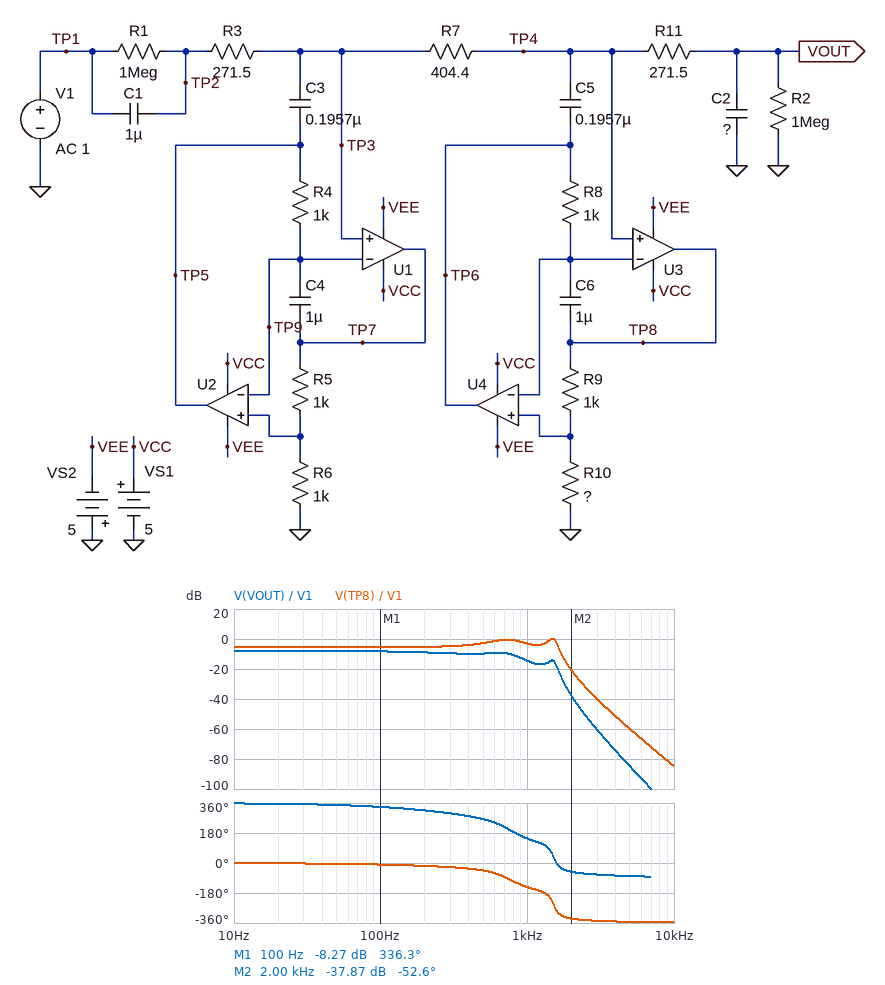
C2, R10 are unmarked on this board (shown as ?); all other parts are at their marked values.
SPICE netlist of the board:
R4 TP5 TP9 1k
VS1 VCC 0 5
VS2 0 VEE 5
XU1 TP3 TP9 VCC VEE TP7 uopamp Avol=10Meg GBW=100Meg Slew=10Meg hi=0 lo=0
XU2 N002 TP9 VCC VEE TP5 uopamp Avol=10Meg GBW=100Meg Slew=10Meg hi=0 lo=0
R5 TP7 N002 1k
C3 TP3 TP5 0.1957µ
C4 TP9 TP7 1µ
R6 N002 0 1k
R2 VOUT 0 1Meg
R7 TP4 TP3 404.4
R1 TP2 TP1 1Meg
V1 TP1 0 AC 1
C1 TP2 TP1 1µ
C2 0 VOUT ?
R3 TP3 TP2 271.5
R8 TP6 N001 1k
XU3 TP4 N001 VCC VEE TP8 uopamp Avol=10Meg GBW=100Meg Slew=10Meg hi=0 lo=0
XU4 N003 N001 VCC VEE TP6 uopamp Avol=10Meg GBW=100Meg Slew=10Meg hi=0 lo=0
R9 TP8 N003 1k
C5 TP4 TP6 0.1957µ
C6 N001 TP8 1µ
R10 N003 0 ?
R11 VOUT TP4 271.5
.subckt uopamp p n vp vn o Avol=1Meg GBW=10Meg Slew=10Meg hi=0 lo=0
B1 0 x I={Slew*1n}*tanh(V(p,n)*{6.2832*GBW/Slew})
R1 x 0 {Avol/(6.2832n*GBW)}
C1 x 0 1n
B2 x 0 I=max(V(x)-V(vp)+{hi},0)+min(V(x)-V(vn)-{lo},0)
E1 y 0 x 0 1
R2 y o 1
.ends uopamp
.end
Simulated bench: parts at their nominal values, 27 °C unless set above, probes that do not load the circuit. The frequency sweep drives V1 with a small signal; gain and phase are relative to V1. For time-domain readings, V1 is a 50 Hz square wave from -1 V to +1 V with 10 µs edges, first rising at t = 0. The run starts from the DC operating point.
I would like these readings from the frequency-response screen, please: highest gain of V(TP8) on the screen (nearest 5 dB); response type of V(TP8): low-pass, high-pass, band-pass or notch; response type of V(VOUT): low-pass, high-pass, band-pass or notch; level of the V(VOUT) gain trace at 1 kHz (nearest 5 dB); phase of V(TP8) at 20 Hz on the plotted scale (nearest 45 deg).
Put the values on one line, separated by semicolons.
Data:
0 dB; low-pass; low-pass; -15 dB; 0 deg
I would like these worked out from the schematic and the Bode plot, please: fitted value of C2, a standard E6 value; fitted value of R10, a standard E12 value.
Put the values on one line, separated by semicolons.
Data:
1.5 µF; 2.7 kΩ
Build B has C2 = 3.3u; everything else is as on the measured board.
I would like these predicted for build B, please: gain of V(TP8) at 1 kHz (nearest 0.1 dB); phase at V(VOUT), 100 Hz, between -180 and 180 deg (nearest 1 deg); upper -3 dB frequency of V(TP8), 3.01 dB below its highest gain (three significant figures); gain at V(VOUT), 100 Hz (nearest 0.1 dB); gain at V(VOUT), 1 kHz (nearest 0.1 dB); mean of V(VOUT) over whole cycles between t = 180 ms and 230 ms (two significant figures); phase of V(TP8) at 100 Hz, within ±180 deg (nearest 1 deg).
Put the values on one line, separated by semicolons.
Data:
-3.2 dB; -27 deg; 1.56 kHz; -13.2 dB; -21.1 dB; -240 mV; 2 deg
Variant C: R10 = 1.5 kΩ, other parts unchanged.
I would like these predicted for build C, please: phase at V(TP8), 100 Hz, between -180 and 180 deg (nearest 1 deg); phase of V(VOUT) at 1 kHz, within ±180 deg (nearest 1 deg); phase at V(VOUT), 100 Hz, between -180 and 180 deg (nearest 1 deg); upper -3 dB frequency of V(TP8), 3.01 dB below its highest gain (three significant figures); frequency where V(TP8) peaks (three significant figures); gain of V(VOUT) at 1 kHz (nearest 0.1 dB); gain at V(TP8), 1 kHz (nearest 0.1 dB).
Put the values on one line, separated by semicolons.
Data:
-10 deg; 128 deg; -25 deg; 1.23 kHz; 1.15 kHz; -10.6 dB; 2.6 dB
